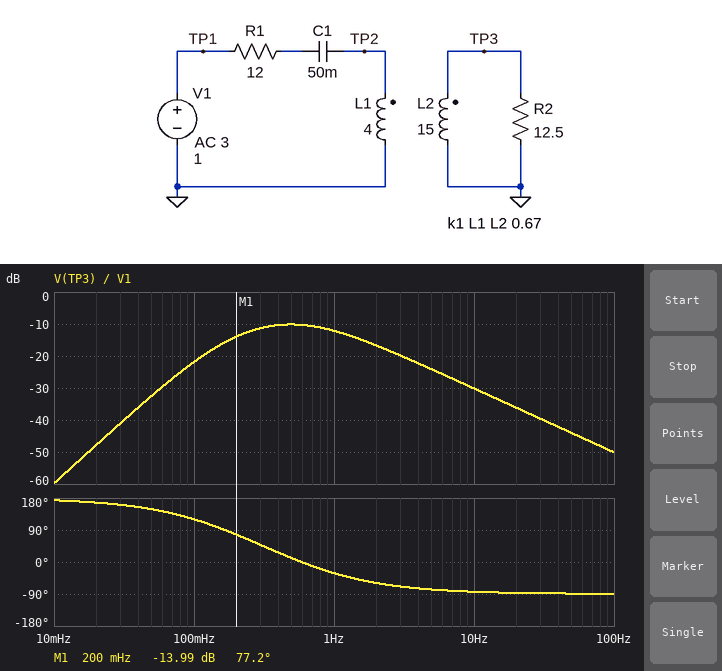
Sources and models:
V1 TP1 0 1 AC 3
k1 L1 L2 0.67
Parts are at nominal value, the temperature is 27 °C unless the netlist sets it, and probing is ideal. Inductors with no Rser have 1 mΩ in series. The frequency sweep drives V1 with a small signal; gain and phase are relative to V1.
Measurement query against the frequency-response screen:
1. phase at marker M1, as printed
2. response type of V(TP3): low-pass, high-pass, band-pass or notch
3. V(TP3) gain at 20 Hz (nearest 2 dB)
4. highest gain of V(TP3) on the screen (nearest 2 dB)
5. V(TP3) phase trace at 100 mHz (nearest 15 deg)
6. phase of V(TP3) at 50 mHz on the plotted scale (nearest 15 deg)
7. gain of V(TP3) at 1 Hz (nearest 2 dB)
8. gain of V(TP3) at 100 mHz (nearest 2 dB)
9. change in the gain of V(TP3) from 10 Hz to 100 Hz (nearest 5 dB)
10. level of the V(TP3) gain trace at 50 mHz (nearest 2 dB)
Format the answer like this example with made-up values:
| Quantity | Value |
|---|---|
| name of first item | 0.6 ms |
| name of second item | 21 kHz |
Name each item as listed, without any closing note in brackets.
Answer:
| Quantity | Value |
|---|---|
| phase at marker M1, as printed | 77.2 deg |
| response type of V(TP3): low-pass, high-pass, band-pass or notch | band-pass |
| V(TP3) gain at 20 Hz | -36 dB |
| highest gain of V(TP3) on the screen | -10 dB |
| V(TP3) phase trace at 100 mHz | 120 deg |
| phase of V(TP3) at 50 mHz on the plotted scale | 150 deg |
| gain of V(TP3) at 1 Hz | -12 dB |
| gain of V(TP3) at 100 mHz | -22 dB |
| change in the gain of V(TP3) from 10 Hz to 100 Hz | -20 dB |
| level of the V(TP3) gain trace at 50 mHz | -32 dB |
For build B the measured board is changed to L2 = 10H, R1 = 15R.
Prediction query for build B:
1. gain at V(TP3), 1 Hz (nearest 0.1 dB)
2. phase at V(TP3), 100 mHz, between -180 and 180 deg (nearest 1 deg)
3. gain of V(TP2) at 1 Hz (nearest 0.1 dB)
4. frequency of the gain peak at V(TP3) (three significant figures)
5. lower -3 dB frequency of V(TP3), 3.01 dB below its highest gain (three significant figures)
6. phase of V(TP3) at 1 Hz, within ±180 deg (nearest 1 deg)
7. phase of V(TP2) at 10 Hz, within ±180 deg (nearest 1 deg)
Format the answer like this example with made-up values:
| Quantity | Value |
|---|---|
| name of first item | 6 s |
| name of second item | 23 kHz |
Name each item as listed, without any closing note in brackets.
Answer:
| Quantity | Value |
|---|---|
| gain at V(TP3), 1 Hz | -11.9 dB |
| phase at V(TP3), 100 mHz, between -180 and 180 deg | 126 deg |
| gain of V(TP2) at 1 Hz | -3.0 dB |
| frequency of the gain peak at V(TP3) | 533 mHz |
| lower -3 dB frequency of V(TP3), 3.01 dB below its highest gain | 221 mHz |
| phase of V(TP3) at 1 Hz, within ±180 deg | -22 deg |
| phase of V(TP2) at 10 Hz, within ±180 deg | 6 deg |
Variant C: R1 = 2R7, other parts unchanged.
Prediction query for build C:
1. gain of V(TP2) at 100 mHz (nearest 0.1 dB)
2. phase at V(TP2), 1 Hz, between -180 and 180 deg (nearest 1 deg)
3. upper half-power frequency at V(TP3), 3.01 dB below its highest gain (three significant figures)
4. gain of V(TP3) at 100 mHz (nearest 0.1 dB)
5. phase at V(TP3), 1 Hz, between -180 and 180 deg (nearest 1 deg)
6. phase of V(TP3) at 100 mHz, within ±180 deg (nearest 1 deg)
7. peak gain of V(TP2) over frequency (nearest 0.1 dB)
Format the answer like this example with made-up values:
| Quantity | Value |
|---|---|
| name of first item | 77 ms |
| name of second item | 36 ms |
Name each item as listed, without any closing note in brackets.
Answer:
| Quantity | Value |
|---|---|
| gain of V(TP2) at 100 mHz | -22.8 dB |
| phase at V(TP2), 1 Hz, between -180 and 180 deg | 15 deg |
| upper half-power frequency at V(TP3), 3.01 dB below its highest gain | 640 mHz |
| gain of V(TP3) at 100 mHz | -21.2 dB |
| phase at V(TP3), 1 Hz, between -180 and 180 deg | -61 deg |
| phase of V(TP3) at 100 mHz, within ±180 deg | 137 deg |
| peak gain of V(TP2) over frequency | 5.0 dB |
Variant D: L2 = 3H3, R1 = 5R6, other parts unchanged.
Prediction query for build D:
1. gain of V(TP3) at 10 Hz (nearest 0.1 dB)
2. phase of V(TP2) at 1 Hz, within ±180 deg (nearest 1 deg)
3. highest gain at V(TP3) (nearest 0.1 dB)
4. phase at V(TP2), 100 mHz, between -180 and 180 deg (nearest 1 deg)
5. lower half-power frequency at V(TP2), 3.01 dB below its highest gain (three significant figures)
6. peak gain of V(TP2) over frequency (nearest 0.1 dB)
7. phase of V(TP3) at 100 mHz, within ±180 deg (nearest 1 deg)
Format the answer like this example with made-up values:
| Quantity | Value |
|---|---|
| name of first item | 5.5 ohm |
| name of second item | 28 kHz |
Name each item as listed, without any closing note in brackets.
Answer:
| Quantity | Value |
|---|---|
| gain of V(TP3) at 10 Hz | -23.6 dB |
| phase of V(TP2) at 1 Hz, within ±180 deg | 21 deg |
| highest gain at V(TP3) | -3.6 dB |
| phase at V(TP2), 100 mHz, between -180 and 180 deg | 165 deg |
| lower half-power frequency at V(TP2), 3.01 dB below its highest gain | 288 mHz |
| peak gain of V(TP2) over frequency | 1.4 dB |
| phase of V(TP3) at 100 mHz, within ±180 deg | 159 deg |
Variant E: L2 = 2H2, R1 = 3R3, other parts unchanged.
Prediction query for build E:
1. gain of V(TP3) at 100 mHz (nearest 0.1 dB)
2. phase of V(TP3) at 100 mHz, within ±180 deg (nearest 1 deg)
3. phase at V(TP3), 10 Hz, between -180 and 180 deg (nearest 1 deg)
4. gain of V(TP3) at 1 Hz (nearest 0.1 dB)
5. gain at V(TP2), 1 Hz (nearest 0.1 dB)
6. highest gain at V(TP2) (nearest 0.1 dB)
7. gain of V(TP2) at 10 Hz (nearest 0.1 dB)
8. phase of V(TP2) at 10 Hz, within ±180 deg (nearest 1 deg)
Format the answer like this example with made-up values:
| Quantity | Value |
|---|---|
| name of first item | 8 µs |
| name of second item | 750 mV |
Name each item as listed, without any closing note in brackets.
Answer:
| Quantity | Value |
|---|---|
| gain of V(TP3) at 100 mHz | -27.5 dB |
| phase of V(TP3) at 100 mHz, within ±180 deg | 167 deg |
| phase at V(TP3), 10 Hz, between -180 and 180 deg | -79 deg |
| gain of V(TP3) at 1 Hz | -6.7 dB |
| gain at V(TP2), 1 Hz | 0.8 dB |
| highest gain at V(TP2) | 5.4 dB |
| gain of V(TP2) at 10 Hz | 0 dB |
| phase of V(TP2) at 10 Hz, within ±180 deg | 1 deg |
